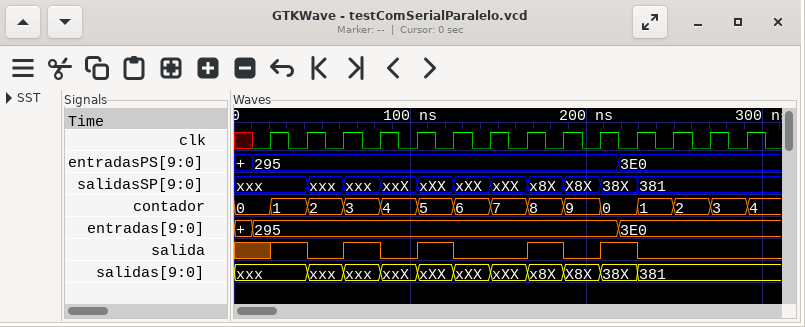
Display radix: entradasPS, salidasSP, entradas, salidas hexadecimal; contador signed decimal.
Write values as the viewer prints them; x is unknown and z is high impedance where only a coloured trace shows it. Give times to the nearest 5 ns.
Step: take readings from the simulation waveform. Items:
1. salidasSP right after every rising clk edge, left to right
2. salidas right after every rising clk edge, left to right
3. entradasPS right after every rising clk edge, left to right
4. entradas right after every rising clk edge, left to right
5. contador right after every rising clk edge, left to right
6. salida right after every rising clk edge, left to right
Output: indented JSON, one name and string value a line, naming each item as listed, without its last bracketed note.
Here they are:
{
  "salidasSP right after every rising clk edge, left to right": "xxx, xxx, xxx, xxX, xXX, xXX, xXX, x8X, X8X, 38X, 381, 381, 381, 381",
  "salidas right after every rising clk edge, left to right": "xxx, xxx, xxx, xxX, xXX, xXX, xXX, x8X, X8X, 38X, 381, 381, 381, 381",
  "entradasPS right after every rising clk edge, left to right": "295, 295, 295, 295, 295, 295, 295, 295, 295, 295, 3E0, 3E0, 3E0, 3E0",
  "entradas right after every rising clk edge, left to right": "295, 295, 295, 295, 295, 295, 295, 295, 295, 295, 3E0, 3E0, 3E0, 3E0",
  "contador right after every rising clk edge, left to right": "1, 2, 3, 4, 5, 6, 7, 8, 9, 0, 1, 2, 3, 4",
  "salida right after every rising clk edge, left to right": "1 0 1 0 1 0 0 1 0 1 0 0 0 0"
}
